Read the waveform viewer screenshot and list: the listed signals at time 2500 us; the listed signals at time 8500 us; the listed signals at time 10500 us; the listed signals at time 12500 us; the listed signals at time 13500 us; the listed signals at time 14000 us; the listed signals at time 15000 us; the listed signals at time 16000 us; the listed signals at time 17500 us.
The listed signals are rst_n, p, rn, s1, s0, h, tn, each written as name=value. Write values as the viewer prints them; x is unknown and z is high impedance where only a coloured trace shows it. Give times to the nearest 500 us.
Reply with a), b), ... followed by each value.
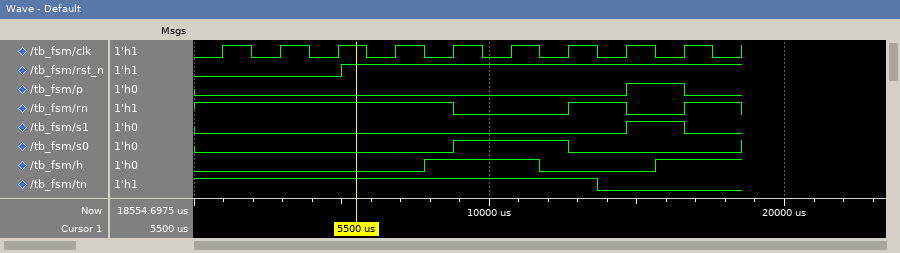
a) rst_n=0, p=0, rn=1, s1=0, s0=0, h=0, tn=1
b) rst_n=1, p=0, rn=1, s1=0, s0=0, h=1, tn=1
c) rst_n=1, p=0, rn=0, s1=0, s0=1, h=1, tn=1
d) rst_n=1, p=0, rn=0, s1=0, s0=1, h=0, tn=1
e) rst_n=1, p=0, rn=1, s1=0, s0=0, h=0, tn=1
f) rst_n=1, p=0, rn=1, s1=0, s0=0, h=0, tn=0
g) rst_n=1, p=1, rn=0, s1=1, s0=0, h=0, tn=0
h) rst_n=1, p=1, rn=0, s1=1, s0=0, h=1, tn=0
i) rst_n=1, p=0, rn=1, s1=0, s0=0, h=1, tn=0
